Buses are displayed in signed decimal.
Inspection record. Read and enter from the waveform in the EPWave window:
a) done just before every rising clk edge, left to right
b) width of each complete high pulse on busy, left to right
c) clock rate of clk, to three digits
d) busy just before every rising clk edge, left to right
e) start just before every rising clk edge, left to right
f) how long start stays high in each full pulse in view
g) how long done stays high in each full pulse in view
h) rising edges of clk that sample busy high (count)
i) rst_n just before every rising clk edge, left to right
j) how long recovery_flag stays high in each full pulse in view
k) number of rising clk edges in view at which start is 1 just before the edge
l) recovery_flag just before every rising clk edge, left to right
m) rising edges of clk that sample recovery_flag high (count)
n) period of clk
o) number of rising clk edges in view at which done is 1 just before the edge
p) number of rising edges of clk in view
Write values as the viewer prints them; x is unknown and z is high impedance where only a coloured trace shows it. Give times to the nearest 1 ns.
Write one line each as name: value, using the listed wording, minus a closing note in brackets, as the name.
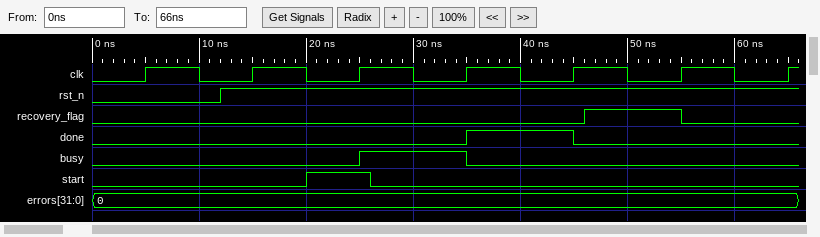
done just before every rising clk edge, left to right: 0 0 0 0 1 0 0
width of each complete high pulse on busy, left to right: 10 ns
clock rate of clk, to three digits: 100 MHz
busy just before every rising clk edge, left to right: 0 0 0 1 0 0 0
start just before every rising clk edge, left to right: 0 0 1 0 0 0 0
how long start stays high in each full pulse in view: 6 ns
how long done stays high in each full pulse in view: 10 ns
rising edges of clk that sample busy high: 1
rst_n just before every rising clk edge, left to right: 0 1 1 1 1 1 1
how long recovery_flag stays high in each full pulse in view: 9 ns
number of rising clk edges in view at which start is 1 just before the edge: 1
recovery_flag just before every rising clk edge, left to right: 0 0 0 0 0 1 0
rising edges of clk that sample recovery_flag high: 1
period of clk: 10 ns
number of rising clk edges in view at which done is 1 just before the edge: 1
number of rising edges of clk in view: 7
